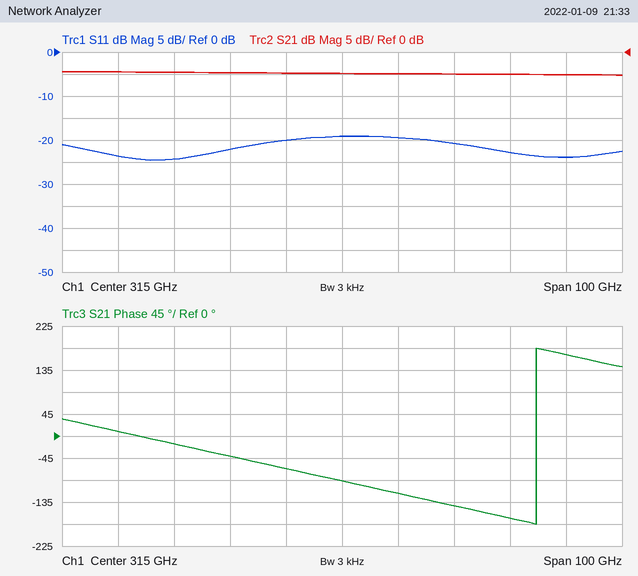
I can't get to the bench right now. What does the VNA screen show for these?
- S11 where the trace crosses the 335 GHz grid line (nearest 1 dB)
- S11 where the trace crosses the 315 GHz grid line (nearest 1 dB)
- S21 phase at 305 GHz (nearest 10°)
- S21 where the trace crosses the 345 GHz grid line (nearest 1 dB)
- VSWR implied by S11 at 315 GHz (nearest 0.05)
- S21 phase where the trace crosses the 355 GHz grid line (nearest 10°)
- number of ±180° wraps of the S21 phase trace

-21 dB
-19 dB
-70°
-5 dB
1.25
170°
1
